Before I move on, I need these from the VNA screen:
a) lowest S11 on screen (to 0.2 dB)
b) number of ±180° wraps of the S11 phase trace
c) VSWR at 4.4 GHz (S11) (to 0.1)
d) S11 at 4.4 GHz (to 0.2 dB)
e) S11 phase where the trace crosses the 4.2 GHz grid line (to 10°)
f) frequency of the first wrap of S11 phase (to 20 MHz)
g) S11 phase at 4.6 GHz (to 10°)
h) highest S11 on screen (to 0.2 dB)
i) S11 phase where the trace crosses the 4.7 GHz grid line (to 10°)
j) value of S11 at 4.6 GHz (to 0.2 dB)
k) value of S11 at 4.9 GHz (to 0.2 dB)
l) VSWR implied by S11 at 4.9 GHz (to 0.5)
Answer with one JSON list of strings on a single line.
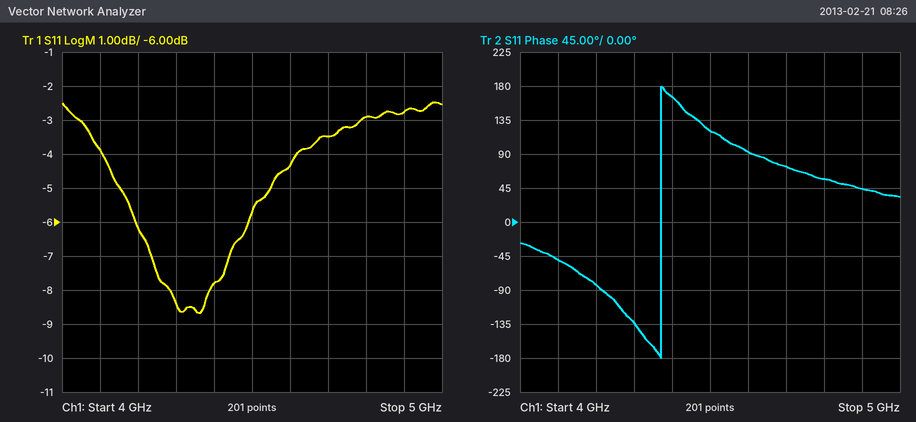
["-8.6 dB", "1", "2.4", "-7.8 dB", "-80°", "4.38 GHz", "90°", "-2.4 dB", "70°", "-4.4 dB", "-2.8 dB", "6.5"]
